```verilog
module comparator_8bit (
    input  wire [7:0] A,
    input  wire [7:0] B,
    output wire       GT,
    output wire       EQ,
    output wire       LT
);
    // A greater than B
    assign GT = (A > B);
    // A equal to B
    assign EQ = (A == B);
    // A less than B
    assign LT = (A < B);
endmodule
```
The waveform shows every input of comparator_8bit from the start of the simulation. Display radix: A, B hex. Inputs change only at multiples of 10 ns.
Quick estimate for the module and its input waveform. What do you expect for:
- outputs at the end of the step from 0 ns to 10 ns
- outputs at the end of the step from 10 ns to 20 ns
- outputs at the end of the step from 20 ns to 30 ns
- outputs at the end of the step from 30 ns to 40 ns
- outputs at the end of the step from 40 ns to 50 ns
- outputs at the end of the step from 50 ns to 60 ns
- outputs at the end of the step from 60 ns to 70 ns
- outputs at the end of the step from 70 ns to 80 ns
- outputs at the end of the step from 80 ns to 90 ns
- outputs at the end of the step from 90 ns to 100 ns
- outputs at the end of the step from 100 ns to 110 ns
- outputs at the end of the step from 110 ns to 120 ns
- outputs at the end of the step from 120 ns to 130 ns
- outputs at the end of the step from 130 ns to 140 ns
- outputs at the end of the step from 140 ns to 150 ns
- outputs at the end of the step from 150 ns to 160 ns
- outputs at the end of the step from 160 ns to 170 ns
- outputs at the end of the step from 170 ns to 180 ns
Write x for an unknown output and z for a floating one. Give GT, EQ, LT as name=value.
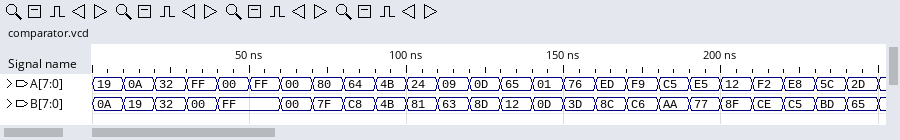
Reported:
GT=1, EQ=0, LT=0
GT=0, EQ=0, LT=1
GT=0, EQ=1, LT=0
GT=1, EQ=0, LT=0
GT=0, EQ=0, LT=1
GT=0, EQ=1, LT=0
GT=0, EQ=1, LT=0
GT=1, EQ=0, LT=0
GT=0, EQ=0, LT=1
GT=0, EQ=1, LT=0
GT=0, EQ=0, LT=1
GT=0, EQ=0, LT=1
GT=0, EQ=0, LT=1
GT=1, EQ=0, LT=0
GT=0, EQ=0, LT=1
GT=1, EQ=0, LT=0
GT=1, EQ=0, LT=0
GT=1, EQ=0, LT=0
